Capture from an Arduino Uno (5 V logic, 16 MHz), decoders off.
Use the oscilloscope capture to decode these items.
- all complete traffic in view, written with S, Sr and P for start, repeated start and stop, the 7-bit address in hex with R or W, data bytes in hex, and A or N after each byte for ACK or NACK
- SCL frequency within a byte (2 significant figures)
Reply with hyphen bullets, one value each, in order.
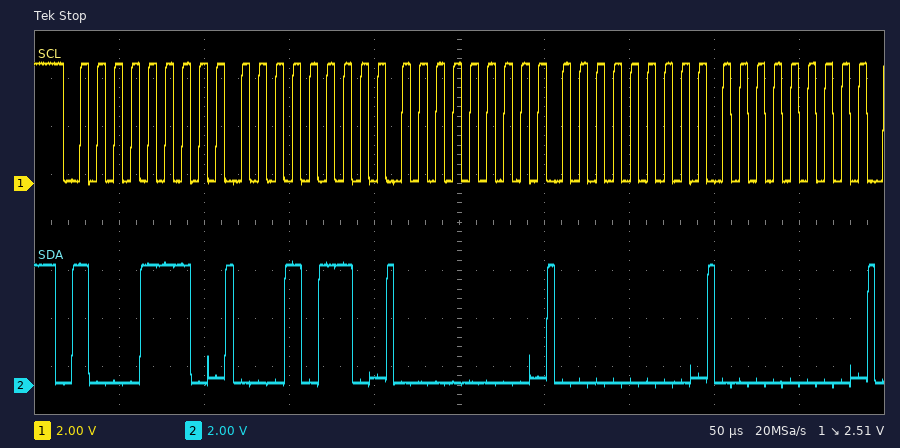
- S 47W A 16 A 00 A 00 A 00 A
- 100 kHz
